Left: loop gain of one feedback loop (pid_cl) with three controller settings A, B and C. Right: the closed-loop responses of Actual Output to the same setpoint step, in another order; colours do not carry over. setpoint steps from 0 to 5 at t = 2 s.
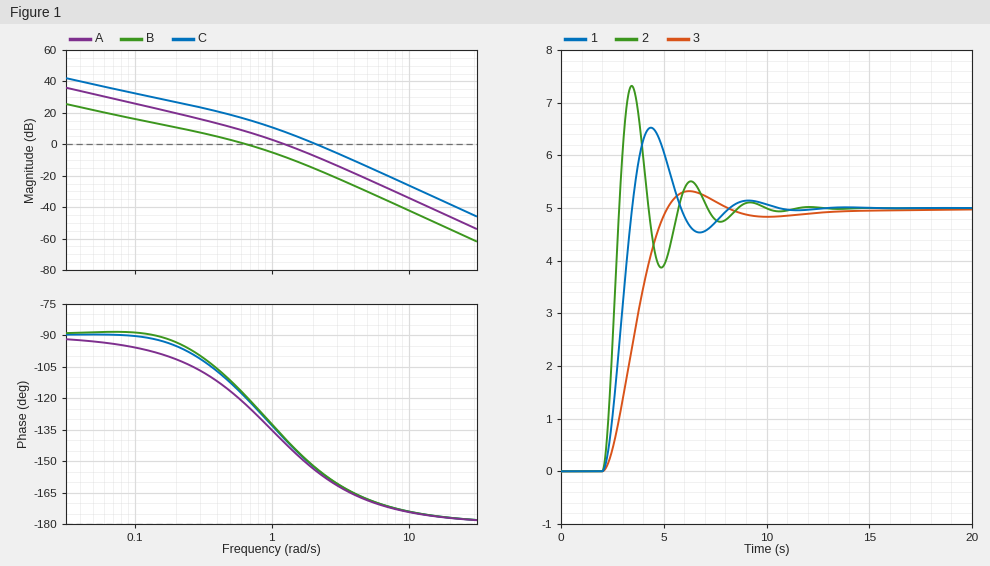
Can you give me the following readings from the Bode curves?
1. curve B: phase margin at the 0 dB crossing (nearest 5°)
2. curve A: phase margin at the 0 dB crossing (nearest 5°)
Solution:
60°
40°
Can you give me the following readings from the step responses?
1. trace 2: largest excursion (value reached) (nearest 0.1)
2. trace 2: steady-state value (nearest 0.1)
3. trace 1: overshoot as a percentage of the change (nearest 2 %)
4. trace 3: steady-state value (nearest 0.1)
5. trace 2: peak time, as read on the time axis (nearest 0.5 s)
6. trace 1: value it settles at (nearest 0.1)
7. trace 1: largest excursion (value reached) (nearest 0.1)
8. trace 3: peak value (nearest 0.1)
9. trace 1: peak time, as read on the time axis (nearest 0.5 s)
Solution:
7.3
5.0
30 %
5.0
3.5 s
5.0
6.5
5.3
4.5 s
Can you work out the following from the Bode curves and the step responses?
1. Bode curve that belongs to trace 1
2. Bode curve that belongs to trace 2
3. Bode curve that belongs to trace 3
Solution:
A
C
B
